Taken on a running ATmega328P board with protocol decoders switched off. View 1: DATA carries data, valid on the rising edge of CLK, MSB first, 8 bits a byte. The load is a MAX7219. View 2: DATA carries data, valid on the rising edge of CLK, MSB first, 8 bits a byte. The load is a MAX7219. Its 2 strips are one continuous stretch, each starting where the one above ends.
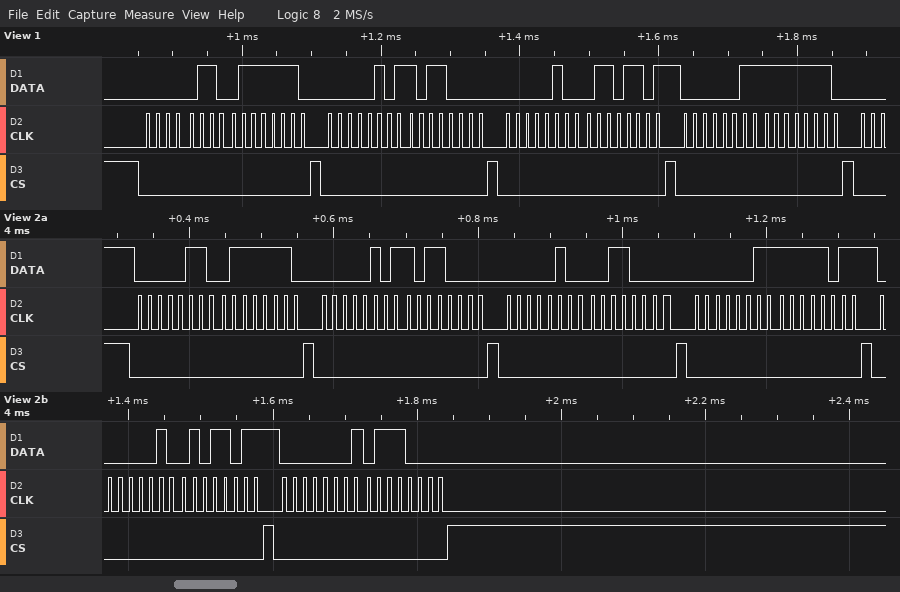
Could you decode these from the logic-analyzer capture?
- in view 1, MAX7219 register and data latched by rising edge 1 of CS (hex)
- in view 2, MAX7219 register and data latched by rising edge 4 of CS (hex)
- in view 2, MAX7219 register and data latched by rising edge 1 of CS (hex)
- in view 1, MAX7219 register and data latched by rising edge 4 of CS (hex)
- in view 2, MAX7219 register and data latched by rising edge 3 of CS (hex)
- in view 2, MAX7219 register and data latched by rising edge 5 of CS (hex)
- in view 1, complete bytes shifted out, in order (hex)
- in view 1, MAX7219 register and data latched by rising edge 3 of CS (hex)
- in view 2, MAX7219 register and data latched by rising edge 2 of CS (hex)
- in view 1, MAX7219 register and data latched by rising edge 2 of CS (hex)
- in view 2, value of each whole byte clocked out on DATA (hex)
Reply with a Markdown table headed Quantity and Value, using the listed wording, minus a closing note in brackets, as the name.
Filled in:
| Quantity | Value |
|---|---|
| in view 1, MAX7219 register and data latched by rising edge 1 of CS | register 0x6, data 0x7E |
| in view 2, MAX7219 register and data latched by rising edge 4 of CS | register 0x3, data 0xFB |
| in view 2, MAX7219 register and data latched by rising edge 1 of CS | register 0x6, data 0x7E |
| in view 1, MAX7219 register and data latched by rising edge 4 of CS | register 0x3, data 0xFE |
| in view 2, MAX7219 register and data latched by rising edge 3 of CS | register 0x4, data 0x30 |
| in view 2, MAX7219 register and data latched by rising edge 5 of CS | register 0x2, data 0x5B |
| in view 1, complete bytes shifted out, in order | 06 7E 05 B0 04 6D 03 FE |
| in view 1, MAX7219 register and data latched by rising edge 3 of CS | register 0x4, data 0x6D |
| in view 2, MAX7219 register and data latched by rising edge 2 of CS | register 0x5, data 0xB0 |
| in view 1, MAX7219 register and data latched by rising edge 2 of CS | register 0x5, data 0xB0 |
| in view 2, value of each whole byte clocked out on DATA | 06 7E 05 B0 04 30 03 FB 02 5B 01 70 |
